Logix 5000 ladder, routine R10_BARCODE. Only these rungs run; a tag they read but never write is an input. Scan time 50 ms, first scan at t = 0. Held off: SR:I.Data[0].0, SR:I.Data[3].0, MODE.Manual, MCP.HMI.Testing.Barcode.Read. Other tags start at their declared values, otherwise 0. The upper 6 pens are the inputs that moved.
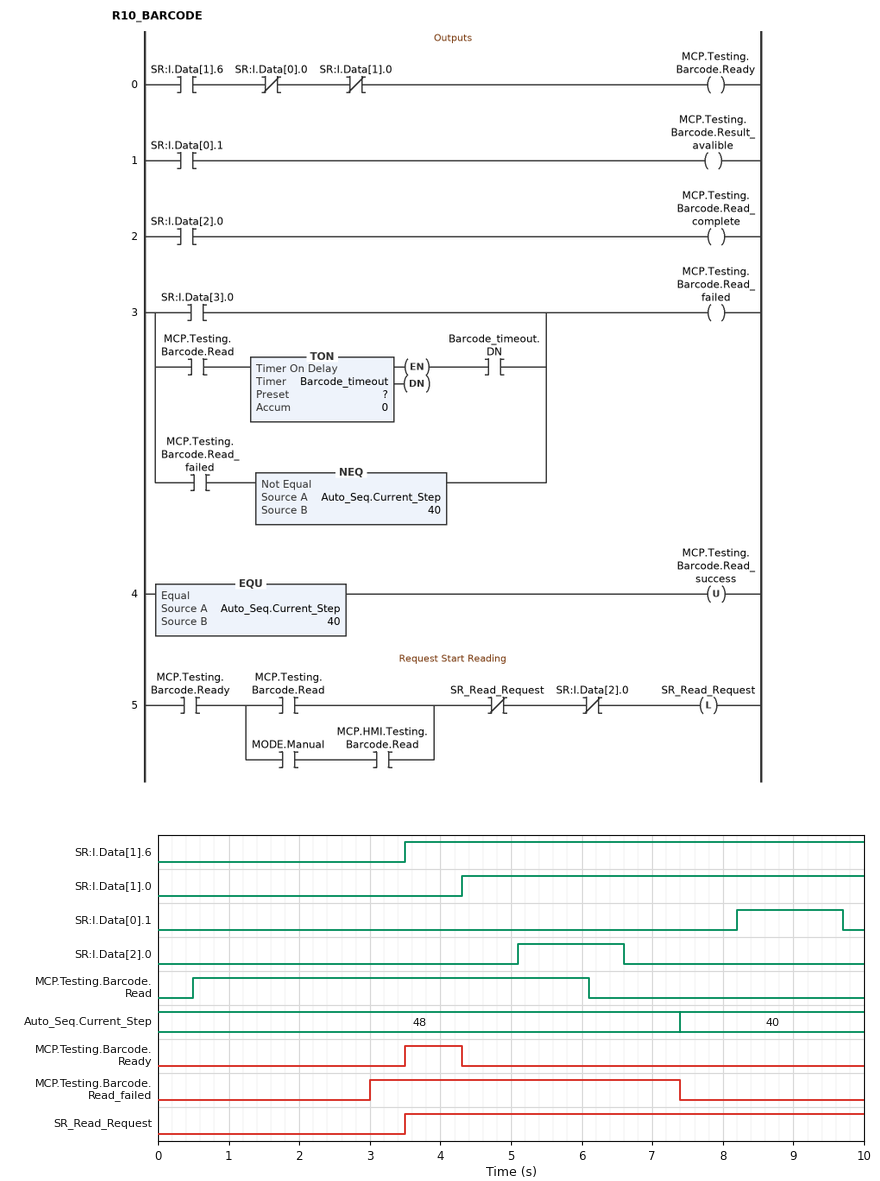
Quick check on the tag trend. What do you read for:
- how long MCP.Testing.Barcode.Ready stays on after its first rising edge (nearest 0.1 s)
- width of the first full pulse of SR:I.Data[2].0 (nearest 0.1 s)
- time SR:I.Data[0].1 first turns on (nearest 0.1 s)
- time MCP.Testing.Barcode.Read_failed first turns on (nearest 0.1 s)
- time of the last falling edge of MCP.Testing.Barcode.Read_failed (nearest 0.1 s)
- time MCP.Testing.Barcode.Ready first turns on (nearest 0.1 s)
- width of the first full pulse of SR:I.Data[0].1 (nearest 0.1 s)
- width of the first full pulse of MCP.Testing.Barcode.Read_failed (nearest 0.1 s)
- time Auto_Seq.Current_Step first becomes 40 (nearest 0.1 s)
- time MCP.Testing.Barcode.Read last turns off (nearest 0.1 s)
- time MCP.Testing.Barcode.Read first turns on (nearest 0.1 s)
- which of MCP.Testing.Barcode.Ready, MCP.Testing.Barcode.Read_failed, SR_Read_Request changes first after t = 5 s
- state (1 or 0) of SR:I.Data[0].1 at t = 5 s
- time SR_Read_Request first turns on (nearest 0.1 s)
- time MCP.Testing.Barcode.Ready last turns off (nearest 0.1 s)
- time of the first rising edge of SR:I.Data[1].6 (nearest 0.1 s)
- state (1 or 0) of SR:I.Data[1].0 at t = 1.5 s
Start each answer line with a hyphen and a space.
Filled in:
- 0.8 s
- 1.5 s
- 8.2 s
- 3.0 s
- 7.4 s
- 3.5 s
- 1.5 s
- 4.4 s
- 7.4 s
- 6.1 s
- 0.5 s
- MCP.Testing.Barcode.Read_failed
- 0
- 3.5 s
- 4.3 s
- 3.5 s
- 0
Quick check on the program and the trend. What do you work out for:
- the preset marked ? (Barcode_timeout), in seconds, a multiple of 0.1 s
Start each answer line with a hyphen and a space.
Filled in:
- 2.5 s
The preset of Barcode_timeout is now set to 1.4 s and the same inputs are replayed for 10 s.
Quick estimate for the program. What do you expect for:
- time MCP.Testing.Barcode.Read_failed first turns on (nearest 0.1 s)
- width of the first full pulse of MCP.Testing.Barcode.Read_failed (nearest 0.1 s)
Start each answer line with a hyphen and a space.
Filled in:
- 1.9 s
- 5.5 s
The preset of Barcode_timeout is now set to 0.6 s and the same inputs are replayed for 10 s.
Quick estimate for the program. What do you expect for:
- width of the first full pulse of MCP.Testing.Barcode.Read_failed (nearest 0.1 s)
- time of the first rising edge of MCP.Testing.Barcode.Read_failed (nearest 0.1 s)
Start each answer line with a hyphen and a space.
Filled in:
- 6.3 s
- 1.1 s
